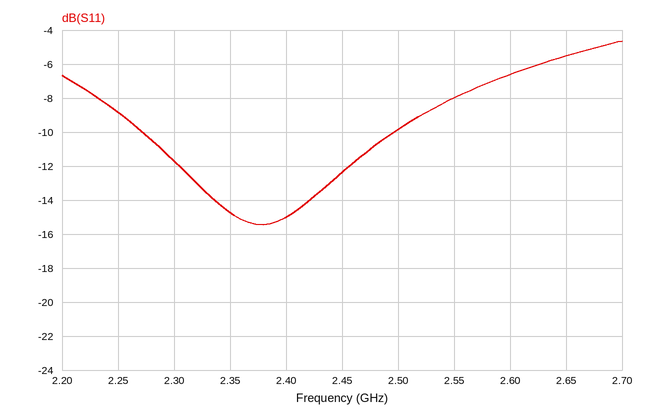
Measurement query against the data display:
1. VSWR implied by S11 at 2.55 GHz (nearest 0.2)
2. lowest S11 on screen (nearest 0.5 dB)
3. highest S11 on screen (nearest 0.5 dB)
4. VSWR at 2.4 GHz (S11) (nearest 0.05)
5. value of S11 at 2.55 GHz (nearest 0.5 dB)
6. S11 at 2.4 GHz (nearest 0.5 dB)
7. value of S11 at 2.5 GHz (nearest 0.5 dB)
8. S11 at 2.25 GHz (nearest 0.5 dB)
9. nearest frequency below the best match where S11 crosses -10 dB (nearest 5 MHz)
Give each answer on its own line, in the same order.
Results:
2.4
-15.5 dB
-4.5 dB
1.45
-8.0 dB
-15.0 dB
-10.0 dB
-9.0 dB
2.270 GHz
